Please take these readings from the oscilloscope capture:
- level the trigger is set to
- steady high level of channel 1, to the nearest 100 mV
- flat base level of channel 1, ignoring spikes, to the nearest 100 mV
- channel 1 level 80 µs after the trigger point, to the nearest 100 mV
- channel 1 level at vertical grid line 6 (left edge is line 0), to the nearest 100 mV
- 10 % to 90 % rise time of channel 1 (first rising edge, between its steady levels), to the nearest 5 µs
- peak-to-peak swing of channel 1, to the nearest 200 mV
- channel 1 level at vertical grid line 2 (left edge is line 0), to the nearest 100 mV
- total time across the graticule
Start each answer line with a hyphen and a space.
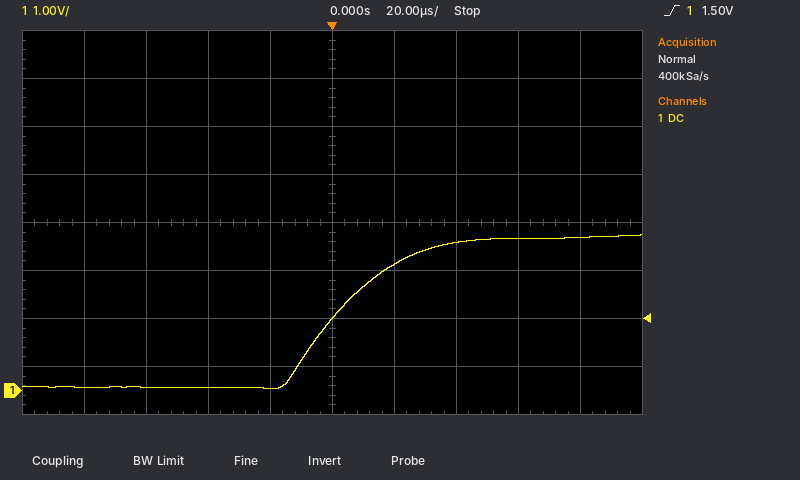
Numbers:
- 1.50 V
- 3.2 V
- 100 mV
- 3.2 V
- 2.6 V
- 40 µs
- 3.2 V
- 100 mV
- 200 µs
